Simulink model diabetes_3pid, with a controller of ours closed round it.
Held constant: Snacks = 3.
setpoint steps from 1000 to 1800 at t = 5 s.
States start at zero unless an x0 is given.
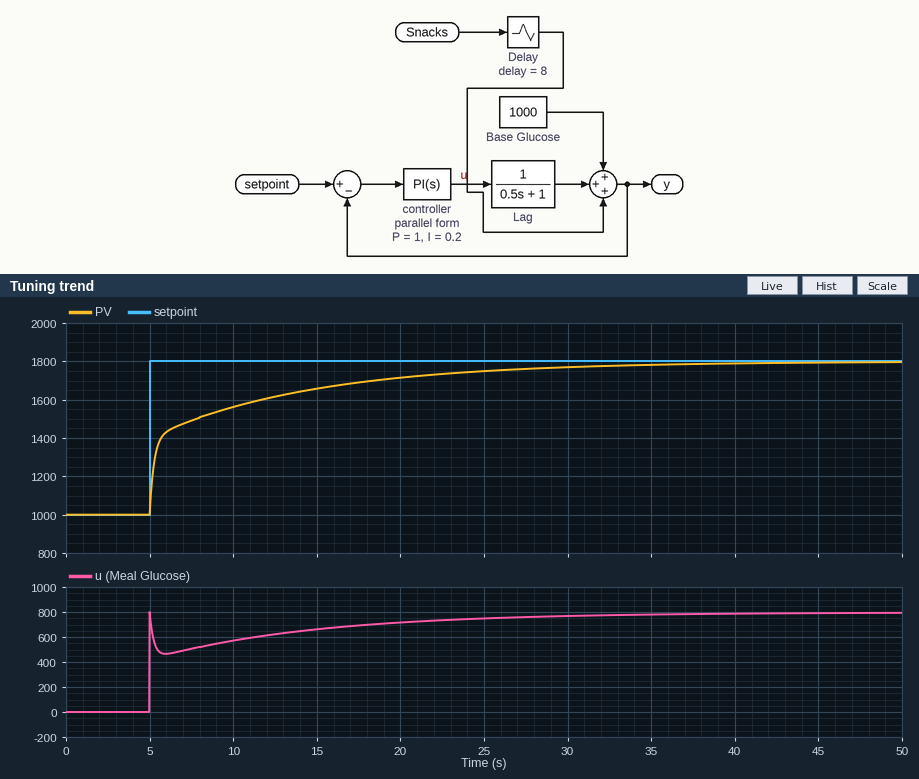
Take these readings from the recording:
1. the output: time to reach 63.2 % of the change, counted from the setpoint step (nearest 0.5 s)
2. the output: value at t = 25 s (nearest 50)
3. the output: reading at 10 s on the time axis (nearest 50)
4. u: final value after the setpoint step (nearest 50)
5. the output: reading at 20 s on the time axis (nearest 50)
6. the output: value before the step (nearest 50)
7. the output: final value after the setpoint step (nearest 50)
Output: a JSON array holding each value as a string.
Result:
["3.0 s", "1750", "1550", "800", "1700", "1000", "1800"]
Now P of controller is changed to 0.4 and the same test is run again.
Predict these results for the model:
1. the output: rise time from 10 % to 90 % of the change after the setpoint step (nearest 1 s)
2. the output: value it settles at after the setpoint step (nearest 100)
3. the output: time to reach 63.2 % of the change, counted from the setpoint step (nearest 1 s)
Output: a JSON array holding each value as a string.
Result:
["13 s", "1800", "5 s"]
